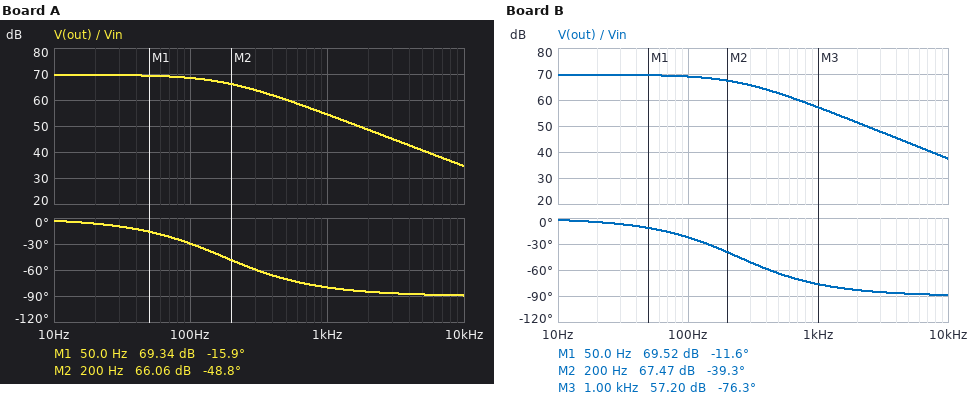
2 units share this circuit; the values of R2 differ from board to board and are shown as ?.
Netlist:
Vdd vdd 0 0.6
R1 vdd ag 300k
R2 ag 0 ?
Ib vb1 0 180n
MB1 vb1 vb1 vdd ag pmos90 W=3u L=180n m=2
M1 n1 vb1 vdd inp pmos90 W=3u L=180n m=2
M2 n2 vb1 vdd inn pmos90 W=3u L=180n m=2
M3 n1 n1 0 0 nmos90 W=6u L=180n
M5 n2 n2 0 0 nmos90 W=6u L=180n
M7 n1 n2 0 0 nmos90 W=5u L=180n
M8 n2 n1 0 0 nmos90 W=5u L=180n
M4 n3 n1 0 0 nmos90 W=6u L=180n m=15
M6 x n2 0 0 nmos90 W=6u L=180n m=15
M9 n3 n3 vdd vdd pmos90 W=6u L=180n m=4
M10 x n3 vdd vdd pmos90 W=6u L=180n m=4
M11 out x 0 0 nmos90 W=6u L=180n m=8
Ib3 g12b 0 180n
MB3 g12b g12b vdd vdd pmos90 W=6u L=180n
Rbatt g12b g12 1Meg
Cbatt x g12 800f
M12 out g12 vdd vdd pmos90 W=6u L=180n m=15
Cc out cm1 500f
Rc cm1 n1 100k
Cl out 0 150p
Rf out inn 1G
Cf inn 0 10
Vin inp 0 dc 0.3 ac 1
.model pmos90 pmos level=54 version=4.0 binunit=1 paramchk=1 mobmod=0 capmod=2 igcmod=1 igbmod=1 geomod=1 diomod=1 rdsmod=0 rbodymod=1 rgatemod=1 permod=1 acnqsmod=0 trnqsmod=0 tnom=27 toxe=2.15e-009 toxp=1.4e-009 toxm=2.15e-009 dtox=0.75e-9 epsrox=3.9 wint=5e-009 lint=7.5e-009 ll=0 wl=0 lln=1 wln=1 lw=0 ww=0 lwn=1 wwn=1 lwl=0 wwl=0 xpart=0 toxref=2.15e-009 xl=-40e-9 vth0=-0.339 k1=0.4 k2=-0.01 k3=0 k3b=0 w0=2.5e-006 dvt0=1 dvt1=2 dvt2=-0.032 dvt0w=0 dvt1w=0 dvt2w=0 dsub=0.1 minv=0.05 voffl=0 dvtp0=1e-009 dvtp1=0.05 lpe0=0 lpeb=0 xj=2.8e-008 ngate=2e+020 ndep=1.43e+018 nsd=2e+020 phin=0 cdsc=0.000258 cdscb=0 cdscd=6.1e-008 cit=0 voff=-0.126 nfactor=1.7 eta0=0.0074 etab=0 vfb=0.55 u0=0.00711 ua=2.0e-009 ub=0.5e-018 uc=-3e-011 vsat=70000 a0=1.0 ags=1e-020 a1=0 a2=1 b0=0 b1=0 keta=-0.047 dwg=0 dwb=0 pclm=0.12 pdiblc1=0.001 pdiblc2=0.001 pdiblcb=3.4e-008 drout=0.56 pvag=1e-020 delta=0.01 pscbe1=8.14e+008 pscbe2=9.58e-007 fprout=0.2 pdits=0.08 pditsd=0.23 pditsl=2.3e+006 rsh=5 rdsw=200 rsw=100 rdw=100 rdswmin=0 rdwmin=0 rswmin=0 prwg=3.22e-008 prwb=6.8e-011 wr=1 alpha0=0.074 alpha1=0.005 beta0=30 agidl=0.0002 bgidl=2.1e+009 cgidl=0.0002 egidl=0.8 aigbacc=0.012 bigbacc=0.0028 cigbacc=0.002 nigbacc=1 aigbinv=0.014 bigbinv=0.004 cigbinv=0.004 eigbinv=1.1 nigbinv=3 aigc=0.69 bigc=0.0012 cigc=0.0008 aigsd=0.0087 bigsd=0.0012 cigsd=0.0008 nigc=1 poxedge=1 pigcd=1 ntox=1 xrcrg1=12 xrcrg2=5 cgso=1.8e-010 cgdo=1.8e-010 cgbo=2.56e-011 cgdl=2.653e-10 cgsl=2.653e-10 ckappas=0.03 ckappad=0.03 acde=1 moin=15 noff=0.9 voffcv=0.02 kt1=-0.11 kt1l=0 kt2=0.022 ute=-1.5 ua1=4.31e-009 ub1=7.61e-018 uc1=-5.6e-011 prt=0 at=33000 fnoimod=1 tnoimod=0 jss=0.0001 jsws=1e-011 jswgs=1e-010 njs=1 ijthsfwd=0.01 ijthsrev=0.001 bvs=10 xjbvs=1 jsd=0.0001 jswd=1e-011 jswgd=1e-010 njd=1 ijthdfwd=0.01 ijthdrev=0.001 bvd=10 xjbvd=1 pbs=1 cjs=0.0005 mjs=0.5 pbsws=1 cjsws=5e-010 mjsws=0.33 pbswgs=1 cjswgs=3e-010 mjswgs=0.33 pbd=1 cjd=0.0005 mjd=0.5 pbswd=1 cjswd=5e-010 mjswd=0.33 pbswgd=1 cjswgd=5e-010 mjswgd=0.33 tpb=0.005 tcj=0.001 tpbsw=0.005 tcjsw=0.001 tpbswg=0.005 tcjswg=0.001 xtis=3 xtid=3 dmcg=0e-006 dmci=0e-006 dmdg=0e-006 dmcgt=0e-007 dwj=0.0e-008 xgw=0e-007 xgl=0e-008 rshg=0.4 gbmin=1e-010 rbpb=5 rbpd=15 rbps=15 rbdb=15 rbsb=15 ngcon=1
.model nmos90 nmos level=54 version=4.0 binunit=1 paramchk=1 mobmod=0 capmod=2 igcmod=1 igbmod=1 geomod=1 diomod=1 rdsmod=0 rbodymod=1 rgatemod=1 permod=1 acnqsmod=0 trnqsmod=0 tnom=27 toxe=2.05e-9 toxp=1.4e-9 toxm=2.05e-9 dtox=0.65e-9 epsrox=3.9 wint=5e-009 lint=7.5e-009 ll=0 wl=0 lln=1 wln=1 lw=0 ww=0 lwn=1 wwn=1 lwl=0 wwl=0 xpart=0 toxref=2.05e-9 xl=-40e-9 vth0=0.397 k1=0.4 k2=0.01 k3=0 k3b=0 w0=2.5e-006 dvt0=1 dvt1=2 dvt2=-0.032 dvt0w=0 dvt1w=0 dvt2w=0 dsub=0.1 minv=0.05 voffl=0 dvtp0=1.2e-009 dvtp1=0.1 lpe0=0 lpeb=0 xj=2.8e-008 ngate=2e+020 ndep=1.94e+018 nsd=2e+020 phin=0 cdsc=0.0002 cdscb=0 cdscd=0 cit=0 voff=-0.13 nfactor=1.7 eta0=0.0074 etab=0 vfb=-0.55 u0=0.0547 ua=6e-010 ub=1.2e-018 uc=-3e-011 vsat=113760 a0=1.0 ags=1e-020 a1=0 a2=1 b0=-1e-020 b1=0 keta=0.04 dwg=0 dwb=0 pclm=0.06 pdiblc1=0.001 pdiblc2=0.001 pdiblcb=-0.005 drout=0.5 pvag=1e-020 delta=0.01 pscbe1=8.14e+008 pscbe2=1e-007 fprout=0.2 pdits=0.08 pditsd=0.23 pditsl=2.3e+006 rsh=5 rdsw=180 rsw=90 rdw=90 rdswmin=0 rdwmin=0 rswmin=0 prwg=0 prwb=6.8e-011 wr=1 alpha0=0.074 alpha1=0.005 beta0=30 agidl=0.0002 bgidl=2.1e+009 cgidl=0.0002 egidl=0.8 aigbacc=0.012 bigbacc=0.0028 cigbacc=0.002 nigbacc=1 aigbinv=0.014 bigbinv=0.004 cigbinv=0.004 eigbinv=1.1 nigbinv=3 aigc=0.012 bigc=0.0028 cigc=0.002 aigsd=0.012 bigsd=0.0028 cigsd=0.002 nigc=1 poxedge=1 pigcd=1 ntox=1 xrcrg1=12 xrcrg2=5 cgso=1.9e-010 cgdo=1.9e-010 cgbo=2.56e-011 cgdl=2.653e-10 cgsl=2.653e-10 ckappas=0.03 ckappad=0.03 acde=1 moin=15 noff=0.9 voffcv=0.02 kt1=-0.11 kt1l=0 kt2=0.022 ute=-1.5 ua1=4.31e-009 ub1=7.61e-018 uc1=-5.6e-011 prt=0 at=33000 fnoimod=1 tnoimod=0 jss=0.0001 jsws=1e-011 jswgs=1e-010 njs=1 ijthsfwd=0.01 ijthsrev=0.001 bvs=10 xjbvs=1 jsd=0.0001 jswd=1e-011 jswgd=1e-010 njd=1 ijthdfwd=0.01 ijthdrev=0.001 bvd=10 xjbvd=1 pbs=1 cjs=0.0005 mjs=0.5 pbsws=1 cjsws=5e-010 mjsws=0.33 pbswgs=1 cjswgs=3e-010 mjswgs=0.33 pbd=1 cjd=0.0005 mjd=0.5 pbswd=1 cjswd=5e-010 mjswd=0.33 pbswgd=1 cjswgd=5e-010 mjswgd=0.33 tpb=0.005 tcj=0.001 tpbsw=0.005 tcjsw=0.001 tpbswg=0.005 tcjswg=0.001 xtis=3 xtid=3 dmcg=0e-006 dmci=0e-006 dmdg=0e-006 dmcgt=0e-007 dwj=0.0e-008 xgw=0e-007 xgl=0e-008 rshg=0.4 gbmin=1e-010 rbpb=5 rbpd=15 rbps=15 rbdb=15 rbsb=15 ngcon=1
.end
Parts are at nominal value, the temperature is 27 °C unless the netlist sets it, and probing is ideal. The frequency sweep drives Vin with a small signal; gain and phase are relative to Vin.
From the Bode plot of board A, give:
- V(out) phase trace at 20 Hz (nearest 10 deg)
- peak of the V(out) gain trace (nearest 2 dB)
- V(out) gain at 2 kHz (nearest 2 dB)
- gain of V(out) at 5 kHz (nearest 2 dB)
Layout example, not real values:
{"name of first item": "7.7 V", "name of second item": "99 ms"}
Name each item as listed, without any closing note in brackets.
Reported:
{"V(out) phase trace at 20 Hz": "-10 deg", "peak of the V(out) gain trace": "70 dB", "V(out) gain at 2 kHz": "48 dB", "gain of V(out) at 5 kHz": "40 dB"}
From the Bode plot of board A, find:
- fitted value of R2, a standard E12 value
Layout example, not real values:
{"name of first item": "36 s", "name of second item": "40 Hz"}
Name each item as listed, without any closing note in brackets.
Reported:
{"fitted value of R2, a standard E12 value": "470 kΩ"}
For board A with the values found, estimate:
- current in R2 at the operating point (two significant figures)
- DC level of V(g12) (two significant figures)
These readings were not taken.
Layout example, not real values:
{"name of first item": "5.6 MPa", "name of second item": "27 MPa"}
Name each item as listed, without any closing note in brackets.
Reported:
{"current in R2 at the operating point": "780 nA", "DC level of V(g12)": "410 mV"}
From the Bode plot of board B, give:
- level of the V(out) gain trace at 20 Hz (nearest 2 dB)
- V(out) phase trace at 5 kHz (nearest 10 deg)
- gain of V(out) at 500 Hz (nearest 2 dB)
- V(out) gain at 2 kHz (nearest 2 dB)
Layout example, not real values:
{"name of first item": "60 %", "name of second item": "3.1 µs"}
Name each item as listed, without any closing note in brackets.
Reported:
{"level of the V(out) gain trace at 20 Hz": "70 dB", "V(out) phase trace at 5 kHz": "-90 deg", "gain of V(out) at 500 Hz": "62 dB", "V(out) gain at 2 kHz": "52 dB"}
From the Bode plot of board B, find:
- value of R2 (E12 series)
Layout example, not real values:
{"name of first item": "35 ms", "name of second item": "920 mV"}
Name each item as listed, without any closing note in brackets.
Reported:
{"value of R2": "820 kΩ"}
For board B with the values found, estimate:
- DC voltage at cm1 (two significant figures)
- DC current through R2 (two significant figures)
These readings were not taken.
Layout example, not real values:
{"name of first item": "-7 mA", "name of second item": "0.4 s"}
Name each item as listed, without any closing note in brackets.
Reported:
{"DC voltage at cm1": "160 mV", "DC current through R2": "540 nA"}
